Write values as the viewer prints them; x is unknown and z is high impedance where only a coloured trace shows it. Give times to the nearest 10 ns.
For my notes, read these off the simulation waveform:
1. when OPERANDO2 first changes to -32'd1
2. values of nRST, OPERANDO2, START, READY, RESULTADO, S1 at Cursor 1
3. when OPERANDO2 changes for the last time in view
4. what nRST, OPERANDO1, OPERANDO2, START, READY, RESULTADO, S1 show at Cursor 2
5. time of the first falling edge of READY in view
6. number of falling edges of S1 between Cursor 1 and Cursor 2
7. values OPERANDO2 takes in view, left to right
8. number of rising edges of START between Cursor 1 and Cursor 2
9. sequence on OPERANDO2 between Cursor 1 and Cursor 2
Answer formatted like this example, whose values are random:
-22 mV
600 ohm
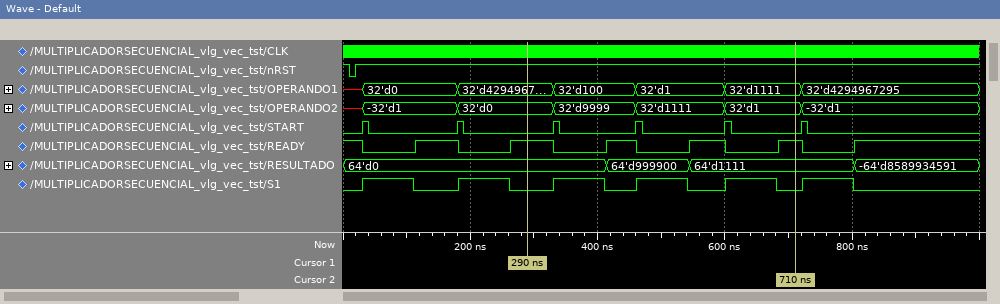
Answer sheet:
30 ns
nRST=1, OPERANDO2=32'd0, START=0, READY=1, RESULTADO=64'd0, S1=0
720 ns
nRST=1, OPERANDO1=32'd1111, OPERANDO2=32'd1, START=0, READY=1, RESULTADO=64'd1111, S1=0
30 ns
3
x, -32'd1, 32'd0, 32'd9999, 32'd1111, 32'd1, -32'd1
3
32'd0, 32'd9999, 32'd1111, 32'd1
